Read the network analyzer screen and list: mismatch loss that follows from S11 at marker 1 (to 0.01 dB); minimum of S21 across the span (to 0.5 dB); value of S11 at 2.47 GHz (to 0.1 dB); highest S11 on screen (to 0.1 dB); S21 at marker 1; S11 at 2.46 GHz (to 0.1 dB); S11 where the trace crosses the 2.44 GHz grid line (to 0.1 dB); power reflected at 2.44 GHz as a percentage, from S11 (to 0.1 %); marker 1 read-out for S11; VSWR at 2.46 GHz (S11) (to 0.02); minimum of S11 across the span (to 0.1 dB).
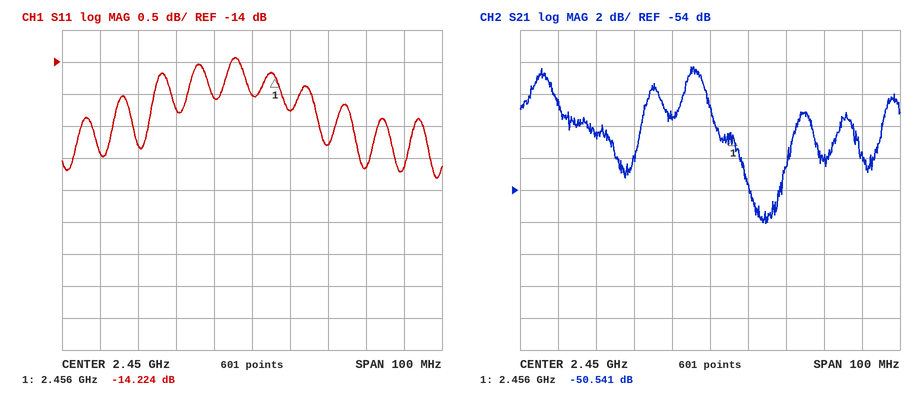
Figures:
0.17 dB
-56.0 dB
-15.3 dB
-13.9 dB
-50.541 dB
-14.8 dB
-14.6 dB
3.5 %
-14.224 dB
1.44
-15.8 dB
